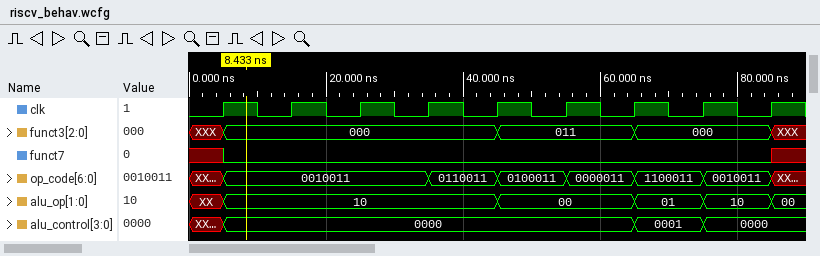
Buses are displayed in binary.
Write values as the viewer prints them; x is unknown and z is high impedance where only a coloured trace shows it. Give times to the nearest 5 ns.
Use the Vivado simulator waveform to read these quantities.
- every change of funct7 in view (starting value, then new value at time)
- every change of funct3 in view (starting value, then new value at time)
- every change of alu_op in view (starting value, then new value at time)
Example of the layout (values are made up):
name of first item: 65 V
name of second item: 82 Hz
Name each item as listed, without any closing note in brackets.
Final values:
every change of funct7 in view: x, 0 at 5 ns, x at 85 ns
every change of funct3 in view: XXX, 000 at 5 ns, 011 at 45 ns, 000 at 65 ns, XXX at 85 ns
every change of alu_op in view: XX, 10 at 5 ns, 00 at 45 ns, 01 at 65 ns, 10 at 75 ns, 00 at 85 ns
